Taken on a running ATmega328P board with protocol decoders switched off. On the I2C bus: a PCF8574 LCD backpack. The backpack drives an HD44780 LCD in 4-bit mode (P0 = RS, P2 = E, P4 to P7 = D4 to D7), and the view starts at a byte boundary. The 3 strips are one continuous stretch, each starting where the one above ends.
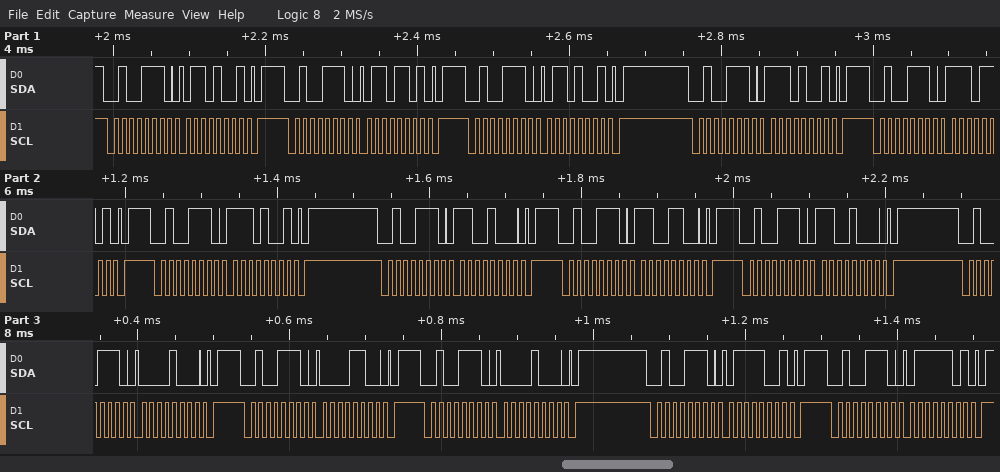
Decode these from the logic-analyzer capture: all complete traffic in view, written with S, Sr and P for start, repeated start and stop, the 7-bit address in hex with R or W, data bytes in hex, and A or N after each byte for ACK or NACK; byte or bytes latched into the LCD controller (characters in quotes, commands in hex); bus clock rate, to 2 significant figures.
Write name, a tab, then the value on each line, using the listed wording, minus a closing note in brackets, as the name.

all complete traffic in view, written with S, Sr and P for start, repeated start and stop, the 7-bit address in hex with R or W, data bytes in hex, and A or N after each byte for ACK or NACK	S 27W A 69 A P S 27W A 6D A P S 27W A 69 A P S 27W A E9 A P S 27W A ED A P S 27W A E9 A P S 27W A C8 A P S 27W A CC A P S 27W A C8 A P S 27W A 08 A P S 27W A 0C A P S 27W A 08 A P S 27W A 79 A P S 27W A 7D A P
byte or bytes latched into the LCD controller	'n' 0xC0
bus clock rate, to 2 significant figures	100 kHz
